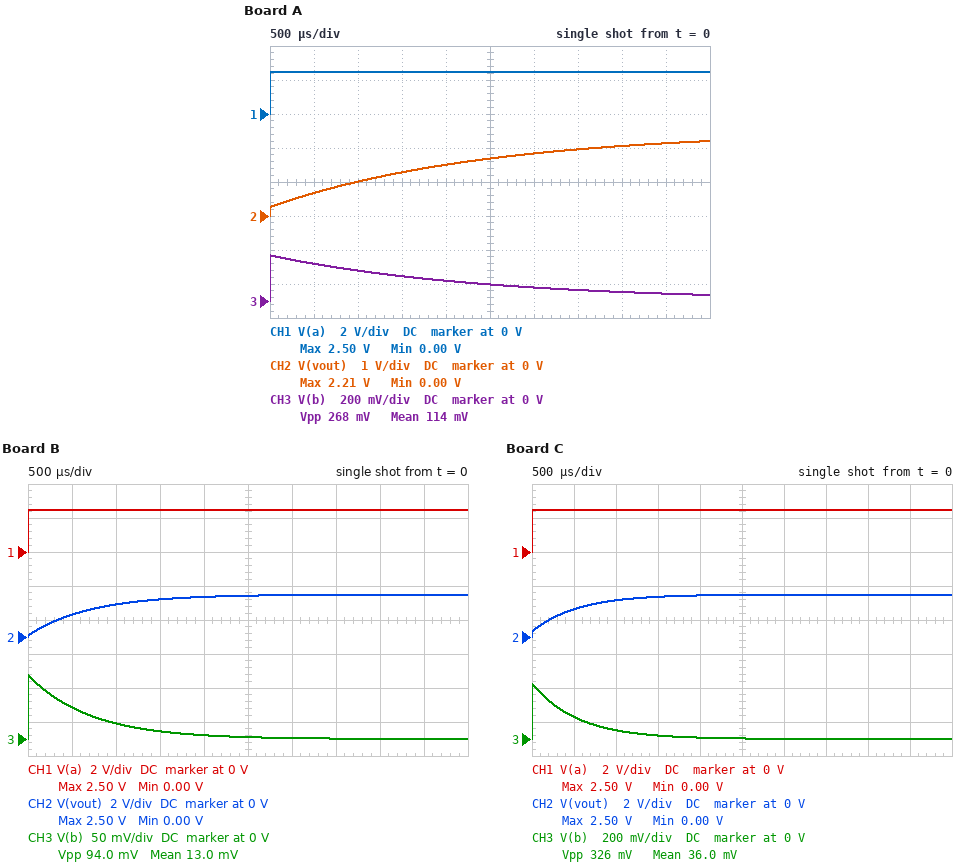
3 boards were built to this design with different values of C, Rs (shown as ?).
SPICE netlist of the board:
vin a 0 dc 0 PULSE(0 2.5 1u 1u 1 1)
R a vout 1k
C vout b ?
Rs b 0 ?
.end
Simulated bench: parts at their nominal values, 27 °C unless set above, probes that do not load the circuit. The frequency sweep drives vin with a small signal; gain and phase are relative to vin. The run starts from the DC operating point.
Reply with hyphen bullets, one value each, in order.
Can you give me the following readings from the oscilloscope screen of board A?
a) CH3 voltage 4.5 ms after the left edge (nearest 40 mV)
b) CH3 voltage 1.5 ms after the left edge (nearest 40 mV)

- 40 mV
- 160 mV
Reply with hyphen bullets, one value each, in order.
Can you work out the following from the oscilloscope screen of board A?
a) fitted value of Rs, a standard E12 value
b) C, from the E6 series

- 120 Ω
- 2.2 µF
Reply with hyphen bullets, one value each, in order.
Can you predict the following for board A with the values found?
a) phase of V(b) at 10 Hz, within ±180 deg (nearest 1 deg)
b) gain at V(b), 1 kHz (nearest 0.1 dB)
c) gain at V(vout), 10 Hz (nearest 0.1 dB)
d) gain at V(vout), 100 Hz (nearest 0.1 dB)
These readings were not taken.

- 81 deg
- -19.4 dB
- -0.1 dB
- -5.2 dB
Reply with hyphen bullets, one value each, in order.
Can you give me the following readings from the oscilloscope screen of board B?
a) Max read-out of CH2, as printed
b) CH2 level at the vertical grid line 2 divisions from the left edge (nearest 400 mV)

- 2.50 V
- 2.0 V
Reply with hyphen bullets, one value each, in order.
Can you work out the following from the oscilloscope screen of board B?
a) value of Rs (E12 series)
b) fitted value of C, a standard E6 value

- 39 Ω
- 680 nF
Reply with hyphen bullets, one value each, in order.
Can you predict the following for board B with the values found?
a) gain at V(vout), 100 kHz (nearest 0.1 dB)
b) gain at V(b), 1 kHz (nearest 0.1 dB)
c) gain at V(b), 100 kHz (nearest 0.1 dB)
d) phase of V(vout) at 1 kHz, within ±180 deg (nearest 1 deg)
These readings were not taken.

- -28.5 dB
- -28.7 dB
- -28.5 dB
- -68 deg
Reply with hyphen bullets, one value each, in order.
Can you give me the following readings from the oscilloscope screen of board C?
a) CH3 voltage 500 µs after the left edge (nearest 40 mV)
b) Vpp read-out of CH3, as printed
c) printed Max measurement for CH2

- 120 mV
- 326 mV
- 2.50 V
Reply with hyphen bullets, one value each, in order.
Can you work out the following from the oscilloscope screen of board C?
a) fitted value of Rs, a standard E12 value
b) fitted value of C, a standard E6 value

- 150 Ω
- 470 nF
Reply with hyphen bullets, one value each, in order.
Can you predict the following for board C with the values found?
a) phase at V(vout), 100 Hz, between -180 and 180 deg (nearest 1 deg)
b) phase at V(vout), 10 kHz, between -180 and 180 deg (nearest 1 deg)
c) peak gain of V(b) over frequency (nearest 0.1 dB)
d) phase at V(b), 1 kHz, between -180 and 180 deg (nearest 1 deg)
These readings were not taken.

- -16 deg
- -11 deg
- -17.7 dB
- 16 deg
